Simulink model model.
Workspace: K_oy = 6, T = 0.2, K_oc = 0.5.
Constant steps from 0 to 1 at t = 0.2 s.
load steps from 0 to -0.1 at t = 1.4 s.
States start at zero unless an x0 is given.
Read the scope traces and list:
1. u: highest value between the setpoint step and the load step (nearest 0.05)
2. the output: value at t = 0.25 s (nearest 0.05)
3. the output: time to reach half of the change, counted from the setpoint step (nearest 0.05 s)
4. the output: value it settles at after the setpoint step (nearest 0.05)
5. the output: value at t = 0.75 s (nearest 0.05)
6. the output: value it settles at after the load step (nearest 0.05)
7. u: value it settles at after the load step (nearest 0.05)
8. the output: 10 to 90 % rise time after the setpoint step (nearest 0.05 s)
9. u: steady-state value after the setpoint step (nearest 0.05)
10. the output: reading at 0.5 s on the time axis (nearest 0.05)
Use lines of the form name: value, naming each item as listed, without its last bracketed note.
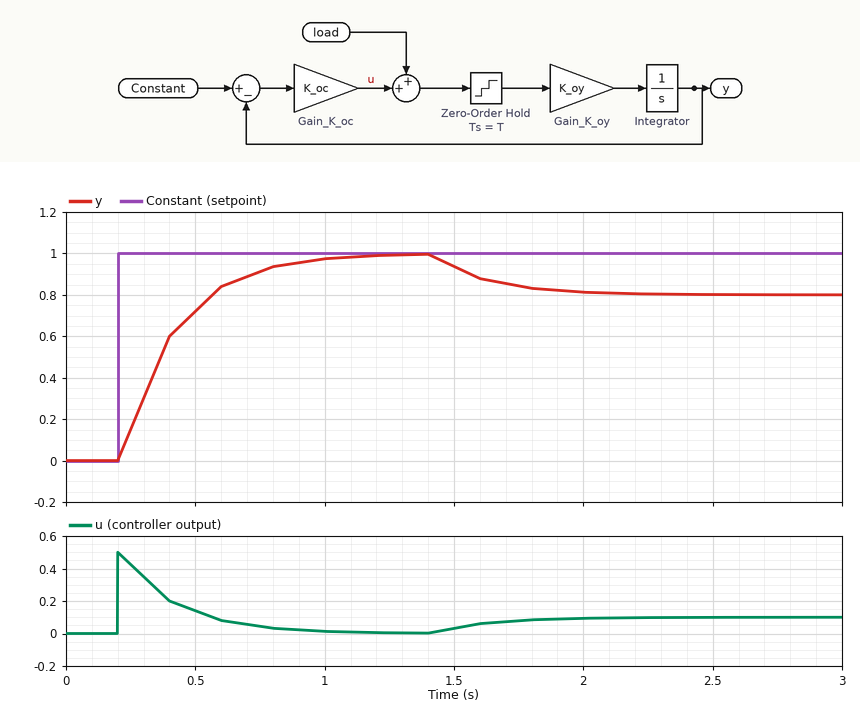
u: highest value between the setpoint step and the load step: 0.50
the output: value at t = 0.25 s: 0.15
the output: time to reach half of the change, counted from the setpoint step: 0.15 s
the output: value it settles at after the setpoint step: 1.00
the output: value at t = 0.75 s: 0.90
the output: value it settles at after the load step: 0.80
u: value it settles at after the load step: 0.10
the output: 10 to 90 % rise time after the setpoint step: 0.50 s
u: steady-state value after the setpoint step: 0.00
the output: reading at 0.5 s on the time axis: 0.70
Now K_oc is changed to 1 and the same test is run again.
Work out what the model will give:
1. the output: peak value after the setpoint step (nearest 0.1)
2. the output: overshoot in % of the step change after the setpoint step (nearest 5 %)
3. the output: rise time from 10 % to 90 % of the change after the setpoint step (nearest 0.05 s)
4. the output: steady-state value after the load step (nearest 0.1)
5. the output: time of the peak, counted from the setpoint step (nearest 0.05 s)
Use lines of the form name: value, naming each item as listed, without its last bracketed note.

the output: peak value after the setpoint step: 1.2
the output: overshoot in % of the step change after the setpoint step: 20 %
the output: rise time from 10 % to 90 % of the change after the setpoint step: 0.15 s
the output: steady-state value after the load step: 0.9
the output: time of the peak, counted from the setpoint step: 0.20 s
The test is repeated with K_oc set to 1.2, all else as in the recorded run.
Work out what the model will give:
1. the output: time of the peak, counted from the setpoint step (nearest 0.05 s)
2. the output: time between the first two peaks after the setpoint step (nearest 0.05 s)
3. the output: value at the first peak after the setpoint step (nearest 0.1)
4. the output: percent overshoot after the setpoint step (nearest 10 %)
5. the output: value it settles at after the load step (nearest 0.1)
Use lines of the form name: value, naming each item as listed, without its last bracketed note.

the output: time of the peak, counted from the setpoint step: 0.20 s
the output: time between the first two peaks after the setpoint step: 0.40 s
the output: value at the first peak after the setpoint step: 1.4
the output: percent overshoot after the setpoint step: 40 %
the output: value it settles at after the load step: 0.9
